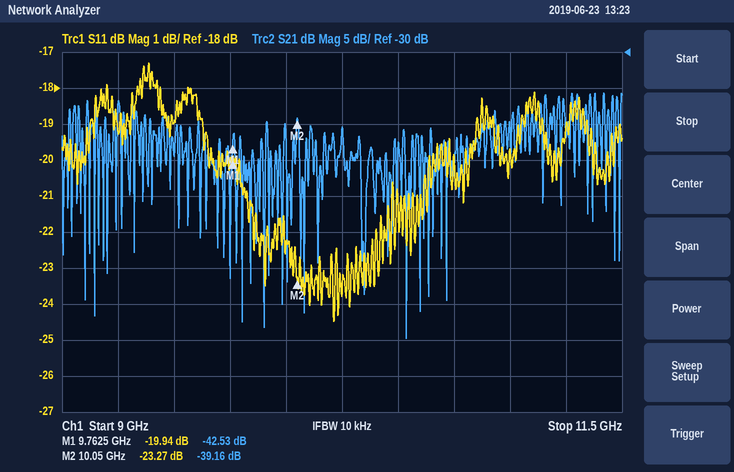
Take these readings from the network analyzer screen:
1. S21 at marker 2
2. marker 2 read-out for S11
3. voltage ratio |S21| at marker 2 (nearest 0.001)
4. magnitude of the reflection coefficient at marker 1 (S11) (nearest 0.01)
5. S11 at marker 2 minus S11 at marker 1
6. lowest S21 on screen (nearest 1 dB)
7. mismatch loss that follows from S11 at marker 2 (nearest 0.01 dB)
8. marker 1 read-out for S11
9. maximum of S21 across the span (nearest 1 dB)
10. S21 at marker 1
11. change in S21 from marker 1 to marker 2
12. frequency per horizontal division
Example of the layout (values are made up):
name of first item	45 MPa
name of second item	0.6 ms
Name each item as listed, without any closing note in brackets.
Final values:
S21 at marker 2	-39.16 dB
marker 2 read-out for S11	-23.27 dB
voltage ratio |S21| at marker 2	0.011
magnitude of the reflection coefficient at marker 1 (S11)	0.10
S11 at marker 2 minus S11 at marker 1	-3.33 dB
lowest S21 on screen	-70 dB
mismatch loss that follows from S11 at marker 2	0.02 dB
marker 1 read-out for S11	-19.94 dB
maximum of S21 across the span	-36 dB
S21 at marker 1	-42.53 dB
change in S21 from marker 1 to marker 2	3.37 dB
frequency per horizontal division	250 MHz
